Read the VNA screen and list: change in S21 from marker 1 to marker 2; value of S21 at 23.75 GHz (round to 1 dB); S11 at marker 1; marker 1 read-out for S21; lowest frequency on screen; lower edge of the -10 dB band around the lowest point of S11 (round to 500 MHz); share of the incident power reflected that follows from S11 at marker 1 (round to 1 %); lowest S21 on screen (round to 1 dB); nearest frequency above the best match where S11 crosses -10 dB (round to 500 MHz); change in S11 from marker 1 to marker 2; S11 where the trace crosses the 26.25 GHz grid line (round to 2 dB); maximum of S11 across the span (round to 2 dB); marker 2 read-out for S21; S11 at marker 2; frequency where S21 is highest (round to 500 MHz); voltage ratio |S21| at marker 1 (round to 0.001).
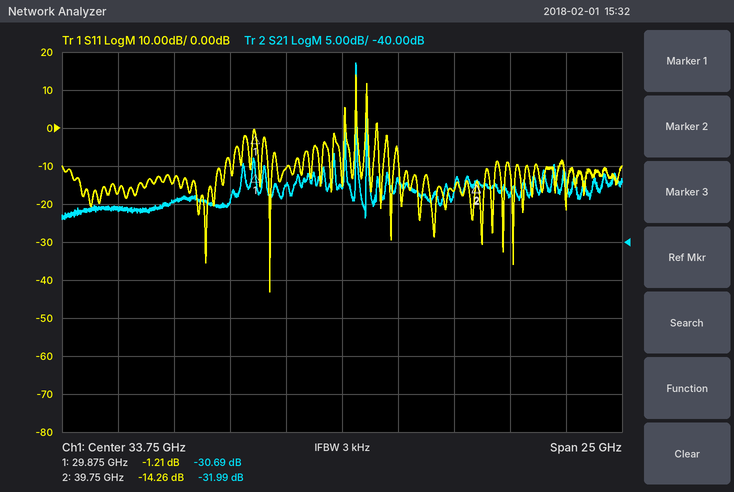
-1.30 dB
-36 dB
-1.21 dB
-30.69 dB
21.25 GHz
30.5 GHz
76 %
-37 dB
30.5 GHz
-13.05 dB
-14 dB
14 dB
-31.99 dB
-14.26 dB
34.5 GHz
0.029
